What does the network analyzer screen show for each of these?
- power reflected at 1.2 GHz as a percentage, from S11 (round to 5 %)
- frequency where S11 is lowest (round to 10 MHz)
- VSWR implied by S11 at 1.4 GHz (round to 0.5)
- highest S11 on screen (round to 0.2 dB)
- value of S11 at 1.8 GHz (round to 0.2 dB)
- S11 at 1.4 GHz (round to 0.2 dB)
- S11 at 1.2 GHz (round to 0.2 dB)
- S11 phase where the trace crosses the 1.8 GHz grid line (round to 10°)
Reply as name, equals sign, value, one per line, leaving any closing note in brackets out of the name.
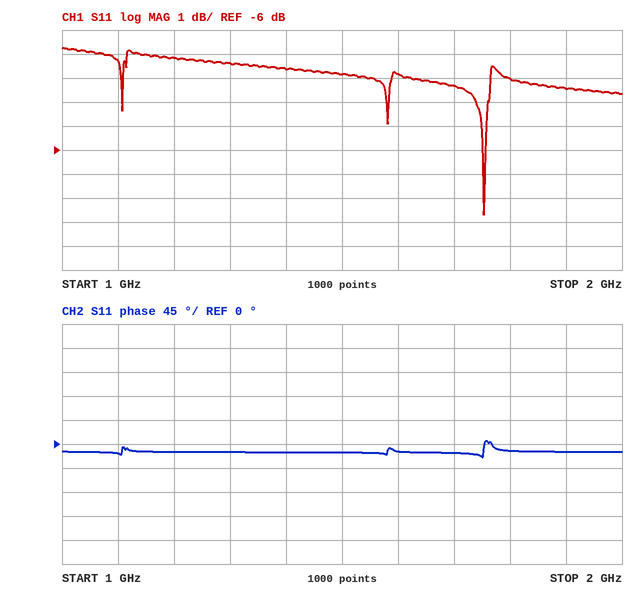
power reflected at 1.2 GHz as a percentage, from S11 = 60 %
frequency where S11 is lowest = 1.75 GHz
VSWR implied by S11 at 1.4 GHz = 6.5
highest S11 on screen = -1.8 dB
value of S11 at 1.8 GHz = -3.0 dB
S11 at 1.4 GHz = -2.6 dB
S11 at 1.2 GHz = -2.2 dB
S11 phase where the trace crosses the 1.8 GHz grid line = -10°
